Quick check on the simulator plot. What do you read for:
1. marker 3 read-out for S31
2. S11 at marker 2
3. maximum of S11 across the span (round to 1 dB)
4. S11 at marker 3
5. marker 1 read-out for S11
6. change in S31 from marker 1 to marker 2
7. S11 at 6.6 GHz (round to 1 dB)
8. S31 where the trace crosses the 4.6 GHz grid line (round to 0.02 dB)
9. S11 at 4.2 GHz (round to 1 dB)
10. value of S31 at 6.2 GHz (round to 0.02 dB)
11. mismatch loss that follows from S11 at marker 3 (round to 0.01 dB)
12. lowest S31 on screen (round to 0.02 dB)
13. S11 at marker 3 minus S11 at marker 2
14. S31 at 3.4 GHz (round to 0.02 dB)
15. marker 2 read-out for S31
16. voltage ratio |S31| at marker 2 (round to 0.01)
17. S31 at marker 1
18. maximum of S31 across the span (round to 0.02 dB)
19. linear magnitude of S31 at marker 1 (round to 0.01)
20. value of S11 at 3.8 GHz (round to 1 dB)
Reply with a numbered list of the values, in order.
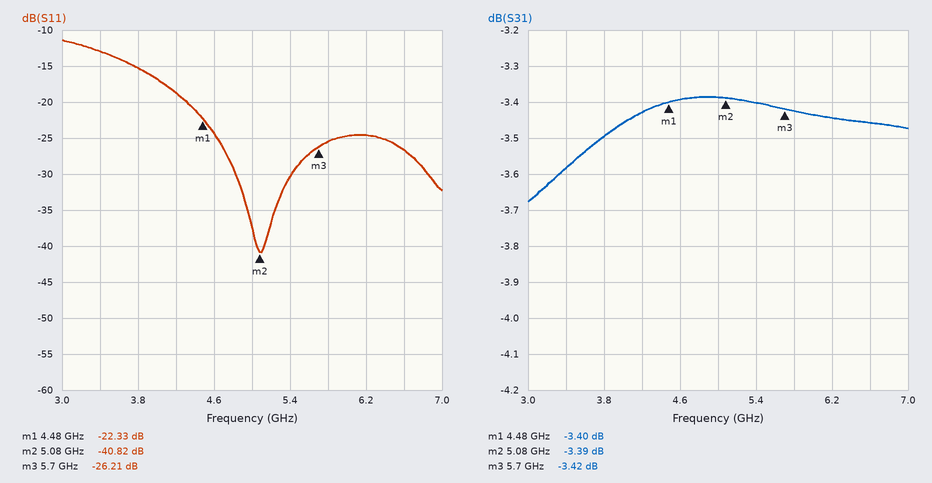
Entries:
1. -3.42 dB
2. -40.82 dB
3. -11 dB
4. -26.21 dB
5. -22.33 dB
6. 0.01 dB
7. -27 dB
8. -3.40 dB
9. -19 dB
10. -3.44 dB
11. 0.01 dB
12. -3.68 dB
13. 14.61 dB
14. -3.58 dB
15. -3.39 dB
16. 0.68
17. -3.40 dB
18. -3.38 dB
19. 0.68
20. -15 dB
